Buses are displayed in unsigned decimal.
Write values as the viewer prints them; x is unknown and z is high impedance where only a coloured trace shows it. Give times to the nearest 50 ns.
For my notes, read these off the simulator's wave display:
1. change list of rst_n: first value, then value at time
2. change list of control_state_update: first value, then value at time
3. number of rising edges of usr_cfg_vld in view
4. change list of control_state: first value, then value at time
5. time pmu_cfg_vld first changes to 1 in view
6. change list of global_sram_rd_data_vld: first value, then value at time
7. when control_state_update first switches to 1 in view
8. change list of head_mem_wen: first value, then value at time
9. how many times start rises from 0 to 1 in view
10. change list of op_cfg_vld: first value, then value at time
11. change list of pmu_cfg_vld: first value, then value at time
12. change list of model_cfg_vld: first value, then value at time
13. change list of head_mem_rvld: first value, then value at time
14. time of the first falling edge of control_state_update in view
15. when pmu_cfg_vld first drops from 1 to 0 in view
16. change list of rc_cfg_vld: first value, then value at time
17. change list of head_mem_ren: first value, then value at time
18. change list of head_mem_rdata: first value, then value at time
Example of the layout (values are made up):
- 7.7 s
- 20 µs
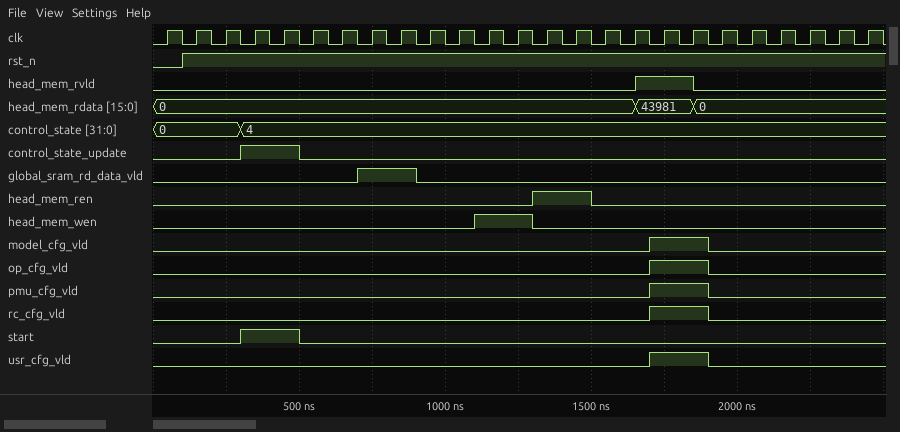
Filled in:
- 0, 1 at 100 ns
- 0, 1 at 300 ns, 0 at 500 ns
- 1
- 0, 4 at 300 ns
- 1700 ns
- 0, 1 at 700 ns, 0 at 900 ns
- 300 ns
- 0, 1 at 1100 ns, 0 at 1300 ns
- 1
- 0, 1 at 1700 ns, 0 at 1900 ns
- 0, 1 at 1700 ns, 0 at 1900 ns
- 0, 1 at 1700 ns, 0 at 1900 ns
- 0, 1 at 1650 ns, 0 at 1850 ns
- 500 ns
- 1900 ns
- 0, 1 at 1700 ns, 0 at 1900 ns
- 0, 1 at 1300 ns, 0 at 1500 ns
- 0, 43981 at 1650 ns, 0 at 1850 ns
